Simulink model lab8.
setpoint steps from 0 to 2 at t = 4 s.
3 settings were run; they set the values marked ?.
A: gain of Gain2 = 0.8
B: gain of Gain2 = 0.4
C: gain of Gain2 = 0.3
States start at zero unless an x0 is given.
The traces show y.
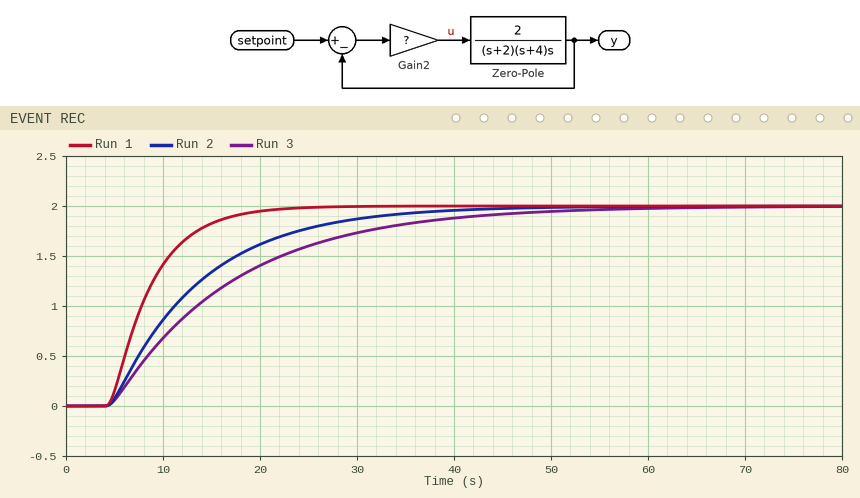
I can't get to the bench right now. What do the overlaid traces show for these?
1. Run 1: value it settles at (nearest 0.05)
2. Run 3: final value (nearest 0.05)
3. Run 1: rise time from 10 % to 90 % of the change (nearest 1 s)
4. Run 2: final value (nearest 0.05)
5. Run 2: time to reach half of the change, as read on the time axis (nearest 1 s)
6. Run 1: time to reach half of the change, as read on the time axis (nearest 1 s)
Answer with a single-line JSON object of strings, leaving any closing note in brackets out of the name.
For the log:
{"Run 1: value it settles at": "2.00", "Run 3: final value": "2.00", "Run 1: rise time from 10 % to 90 % of the change": "9 s", "Run 2: final value": "2.00", "Run 2: time to reach half of the change, as read on the time axis": "11 s", "Run 1: time to reach half of the change, as read on the time axis": "8 s"}
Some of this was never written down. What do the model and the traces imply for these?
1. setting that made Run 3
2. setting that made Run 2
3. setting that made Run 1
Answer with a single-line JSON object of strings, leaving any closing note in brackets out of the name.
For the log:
{"setting that made Run 3": "C", "setting that made Run 2": "B", "setting that made Run 1": "A"}
